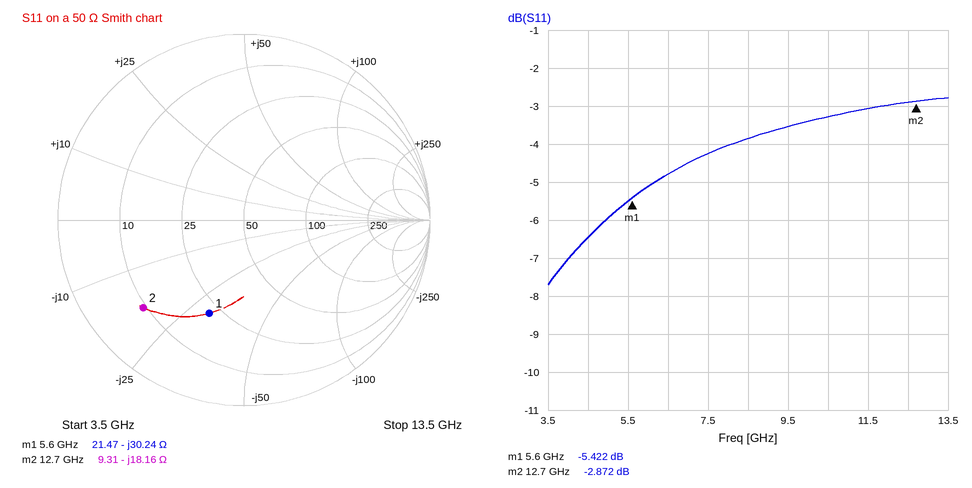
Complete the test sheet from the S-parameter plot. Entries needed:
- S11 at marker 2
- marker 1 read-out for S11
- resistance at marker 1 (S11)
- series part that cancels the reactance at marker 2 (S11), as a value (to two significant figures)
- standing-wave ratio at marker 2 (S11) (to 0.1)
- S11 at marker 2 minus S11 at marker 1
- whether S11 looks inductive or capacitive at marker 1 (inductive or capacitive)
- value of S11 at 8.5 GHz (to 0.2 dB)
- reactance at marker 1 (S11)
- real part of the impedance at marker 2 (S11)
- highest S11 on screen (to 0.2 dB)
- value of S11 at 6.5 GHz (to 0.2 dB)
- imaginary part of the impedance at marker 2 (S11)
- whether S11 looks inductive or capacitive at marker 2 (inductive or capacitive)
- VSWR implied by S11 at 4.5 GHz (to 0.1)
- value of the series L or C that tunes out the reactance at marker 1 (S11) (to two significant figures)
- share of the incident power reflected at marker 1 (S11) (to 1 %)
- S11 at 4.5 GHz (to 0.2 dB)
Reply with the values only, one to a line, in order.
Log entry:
-2.872 dB
-5.422 dB
21.47 Ω
230 pH
6.1
2.550 dB
capacitive
-3.8 dB
-30.24 Ω
9.31 Ω
-2.8 dB
-4.8 dB
-18.16 Ω
capacitive
2.8
860 pH
29 %
-6.4 dB
